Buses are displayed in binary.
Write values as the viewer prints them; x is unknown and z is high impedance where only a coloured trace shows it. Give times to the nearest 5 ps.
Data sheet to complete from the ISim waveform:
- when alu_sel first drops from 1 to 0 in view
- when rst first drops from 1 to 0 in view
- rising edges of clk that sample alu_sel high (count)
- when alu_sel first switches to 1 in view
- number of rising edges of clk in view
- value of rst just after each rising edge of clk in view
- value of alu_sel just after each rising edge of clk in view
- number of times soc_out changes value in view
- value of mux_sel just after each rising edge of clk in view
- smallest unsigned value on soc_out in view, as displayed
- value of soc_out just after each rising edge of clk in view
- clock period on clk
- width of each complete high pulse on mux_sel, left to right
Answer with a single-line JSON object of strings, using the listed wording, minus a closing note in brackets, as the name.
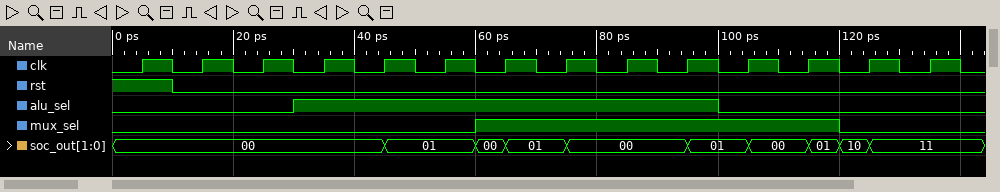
{"when alu_sel first drops from 1 to 0 in view": "100 ps", "when rst first drops from 1 to 0 in view": "10 ps", "rising edges of clk that sample alu_sel high": "7", "when alu_sel first switches to 1 in view": "30 ps", "number of rising edges of clk in view": "14", "value of rst just after each rising edge of clk in view": "1 0 0 0 0 0 0 0 0 0 0 0 0 0", "value of alu_sel just after each rising edge of clk in view": "0 0 0 1 1 1 1 1 1 1 0 0 0 0", "number of times soc_out changes value in view": "9", "value of mux_sel just after each rising edge of clk in view": "0 0 0 0 0 0 1 1 1 1 1 1 0 0", "smallest unsigned value on soc_out in view, as displayed": "00", "value of soc_out just after each rising edge of clk in view": "00, 00, 00, 00, 01, 01, 01, 00, 00, 01, 00, 01, 11, 11", "clock period on clk": "10 ps", "width of each complete high pulse on mux_sel, left to right": "60 ps"}
